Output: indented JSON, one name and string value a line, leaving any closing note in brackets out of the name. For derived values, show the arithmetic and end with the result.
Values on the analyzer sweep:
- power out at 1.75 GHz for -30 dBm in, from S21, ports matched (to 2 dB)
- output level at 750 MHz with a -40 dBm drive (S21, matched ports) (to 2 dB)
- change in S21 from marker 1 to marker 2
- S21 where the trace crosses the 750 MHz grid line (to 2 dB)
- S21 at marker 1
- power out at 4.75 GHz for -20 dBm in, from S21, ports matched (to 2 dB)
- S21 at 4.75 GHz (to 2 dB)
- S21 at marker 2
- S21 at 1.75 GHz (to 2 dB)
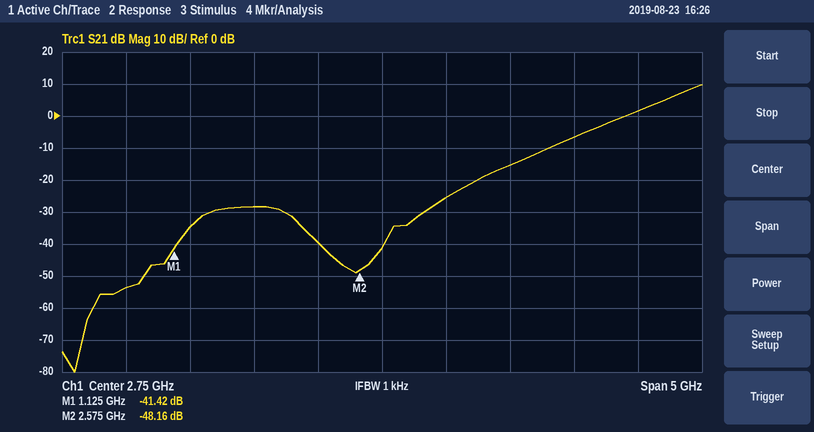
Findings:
{
  "power out at 1.75 GHz for -30 dBm in, from S21, ports matched": "-30 dBm + (-28 dB) = -58 dBm",
  "output level at 750 MHz with a -40 dBm drive (S21, matched ports)": "-40 dBm + (-54 dB) = -94 dBm",
  "change in S21 from marker 1 to marker 2": "-48.16 − (-41.42) = -6.74 dB",
  "S21 where the trace crosses the 750 MHz grid line": "-54 dB",
  "S21 at marker 1": "-41.42 dB",
  "power out at 4.75 GHz for -20 dBm in, from S21, ports matched": "-20 dBm + (2 dB) = -18 dBm",
  "S21 at 4.75 GHz": "2 dB",
  "S21 at marker 2": "-48.16 dB",
  "S21 at 1.75 GHz": "-28 dB"
}
